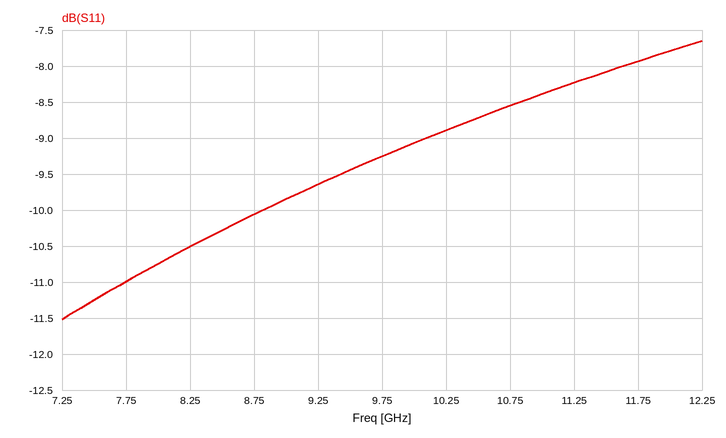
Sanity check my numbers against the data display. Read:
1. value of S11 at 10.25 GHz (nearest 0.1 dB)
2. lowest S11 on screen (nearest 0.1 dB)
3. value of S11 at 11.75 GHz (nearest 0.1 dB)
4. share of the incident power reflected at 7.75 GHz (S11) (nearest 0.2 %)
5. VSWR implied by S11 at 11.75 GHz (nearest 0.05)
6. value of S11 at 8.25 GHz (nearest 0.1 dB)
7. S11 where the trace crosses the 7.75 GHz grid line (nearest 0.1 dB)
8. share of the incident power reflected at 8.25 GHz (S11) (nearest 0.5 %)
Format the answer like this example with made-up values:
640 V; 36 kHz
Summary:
-8.9 dB; -11.5 dB; -7.9 dB; 8.0 %; 2.35; -10.5 dB; -11.0 dB; 9.0 %
